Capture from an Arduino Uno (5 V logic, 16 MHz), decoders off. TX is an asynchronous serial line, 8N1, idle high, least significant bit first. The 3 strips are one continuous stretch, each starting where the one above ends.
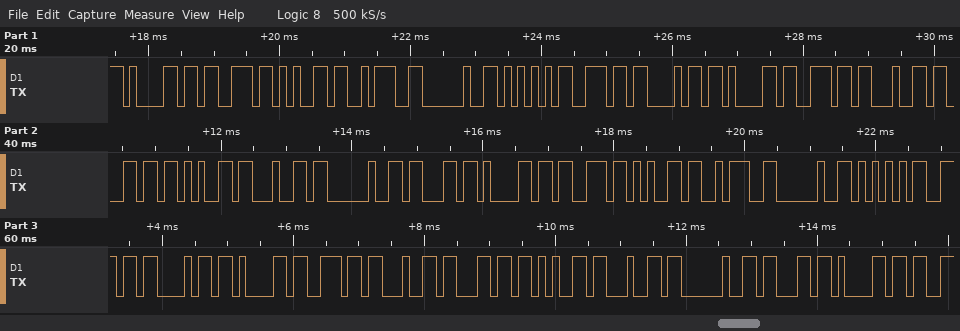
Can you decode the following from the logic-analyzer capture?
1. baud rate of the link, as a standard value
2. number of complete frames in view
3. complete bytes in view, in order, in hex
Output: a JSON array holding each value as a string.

["9600 baud", "33", "61 73 65 3A 20 55 6E 68 61 6E 64 6C 65 64 20 63 61 73 65 3A 20 55 6E 68 61 6E 64 6C 65 64 20 63 61"]
